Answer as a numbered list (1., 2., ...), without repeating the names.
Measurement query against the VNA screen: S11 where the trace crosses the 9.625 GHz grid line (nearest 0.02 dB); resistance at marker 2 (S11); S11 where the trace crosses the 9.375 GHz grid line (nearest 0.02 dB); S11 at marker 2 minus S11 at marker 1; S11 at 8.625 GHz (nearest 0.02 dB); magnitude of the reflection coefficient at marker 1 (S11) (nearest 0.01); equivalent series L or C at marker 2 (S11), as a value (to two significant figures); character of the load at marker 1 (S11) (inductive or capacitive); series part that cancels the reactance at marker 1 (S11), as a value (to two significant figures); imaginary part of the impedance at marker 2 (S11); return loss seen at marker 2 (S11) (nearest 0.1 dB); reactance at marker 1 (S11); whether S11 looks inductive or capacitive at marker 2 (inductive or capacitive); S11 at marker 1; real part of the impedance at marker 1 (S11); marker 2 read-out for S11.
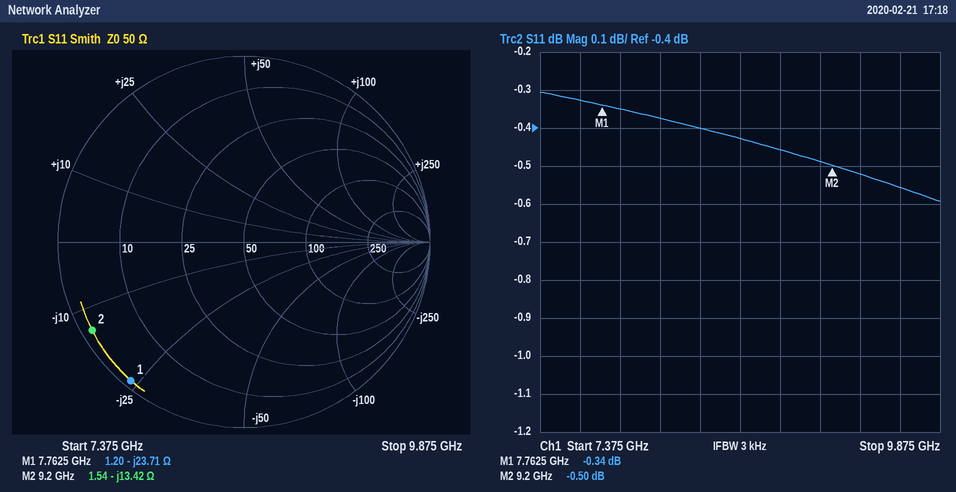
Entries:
1. -0.56 dB
2. 1.54 Ω
3. -0.52 dB
4. -0.16 dB
5. -0.42 dB
6. 0.96
7. 1.3 pF
8. capacitive
9. 490 pH
10. -13.42 Ω
11. 0.5 dB
12. -23.71 Ω
13. capacitive
14. -0.34 dB
15. 1.20 Ω
16. -0.50 dB
